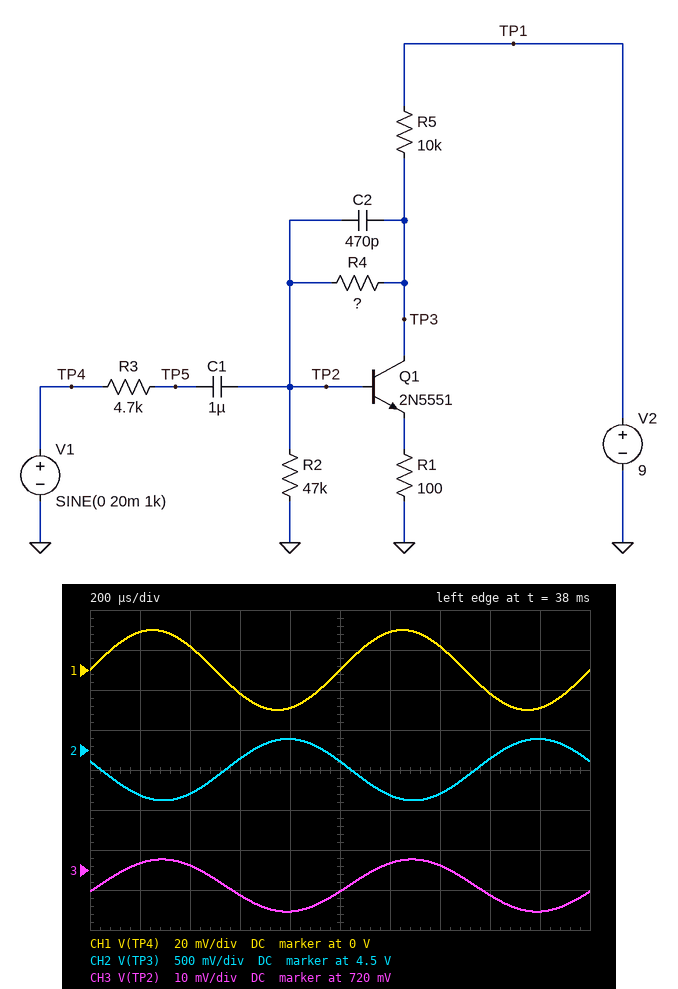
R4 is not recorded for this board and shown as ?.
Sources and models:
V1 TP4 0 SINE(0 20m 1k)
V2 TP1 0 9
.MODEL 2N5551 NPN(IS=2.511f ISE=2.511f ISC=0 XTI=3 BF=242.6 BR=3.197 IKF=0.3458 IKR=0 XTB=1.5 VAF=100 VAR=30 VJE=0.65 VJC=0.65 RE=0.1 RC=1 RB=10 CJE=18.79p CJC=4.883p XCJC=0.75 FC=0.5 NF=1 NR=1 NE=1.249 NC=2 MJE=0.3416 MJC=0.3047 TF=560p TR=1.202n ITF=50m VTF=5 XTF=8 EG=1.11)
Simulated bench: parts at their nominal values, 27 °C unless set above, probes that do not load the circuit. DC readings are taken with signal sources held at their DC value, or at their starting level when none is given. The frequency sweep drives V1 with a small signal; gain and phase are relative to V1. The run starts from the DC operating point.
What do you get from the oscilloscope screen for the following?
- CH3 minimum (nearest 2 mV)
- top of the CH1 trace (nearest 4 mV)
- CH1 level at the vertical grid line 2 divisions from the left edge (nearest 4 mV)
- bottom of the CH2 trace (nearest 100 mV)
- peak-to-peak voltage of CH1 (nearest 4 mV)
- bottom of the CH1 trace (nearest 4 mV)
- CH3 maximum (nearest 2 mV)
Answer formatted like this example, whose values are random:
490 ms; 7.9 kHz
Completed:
710 mV; 20 mV; 12 mV; 3.9 V; 40 mV; -20 mV; 722 mV
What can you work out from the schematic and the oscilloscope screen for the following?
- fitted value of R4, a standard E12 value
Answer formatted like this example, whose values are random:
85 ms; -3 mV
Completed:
180 kΩ
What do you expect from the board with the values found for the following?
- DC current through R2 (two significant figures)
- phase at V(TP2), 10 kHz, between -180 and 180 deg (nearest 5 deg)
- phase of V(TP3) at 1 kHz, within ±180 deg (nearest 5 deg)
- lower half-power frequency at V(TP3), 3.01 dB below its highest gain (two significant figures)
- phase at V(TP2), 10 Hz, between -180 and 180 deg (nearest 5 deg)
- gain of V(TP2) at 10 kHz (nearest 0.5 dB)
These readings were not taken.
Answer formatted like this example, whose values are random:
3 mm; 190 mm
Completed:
15 µA; -55 deg; 165 deg; 22 Hz; 65 deg; -19.0 dB
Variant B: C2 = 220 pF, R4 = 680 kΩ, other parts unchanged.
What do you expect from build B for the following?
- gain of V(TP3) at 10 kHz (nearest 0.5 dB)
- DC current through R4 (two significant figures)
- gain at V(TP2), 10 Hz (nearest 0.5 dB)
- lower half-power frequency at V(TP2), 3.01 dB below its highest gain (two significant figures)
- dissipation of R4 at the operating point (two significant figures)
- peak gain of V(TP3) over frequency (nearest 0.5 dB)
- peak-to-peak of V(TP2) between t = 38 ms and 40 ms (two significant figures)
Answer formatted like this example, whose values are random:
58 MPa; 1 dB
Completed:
7.0 dB; 12 µA; -2.0 dB; 4.3 Hz; 100 µW; 7.5 dB; 35 mV
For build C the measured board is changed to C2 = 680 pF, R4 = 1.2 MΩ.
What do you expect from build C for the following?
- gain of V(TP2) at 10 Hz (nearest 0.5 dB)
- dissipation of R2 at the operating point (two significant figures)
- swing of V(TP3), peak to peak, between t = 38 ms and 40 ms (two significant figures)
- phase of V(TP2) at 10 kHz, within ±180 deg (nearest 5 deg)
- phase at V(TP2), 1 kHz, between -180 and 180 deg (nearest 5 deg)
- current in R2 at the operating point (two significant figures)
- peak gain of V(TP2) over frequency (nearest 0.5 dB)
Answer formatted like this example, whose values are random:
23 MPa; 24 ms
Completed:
-1.5 dB; 2.4 µW; 1.6 mV; -10 deg; 0 deg; 7.2 µA; -1.0 dB
